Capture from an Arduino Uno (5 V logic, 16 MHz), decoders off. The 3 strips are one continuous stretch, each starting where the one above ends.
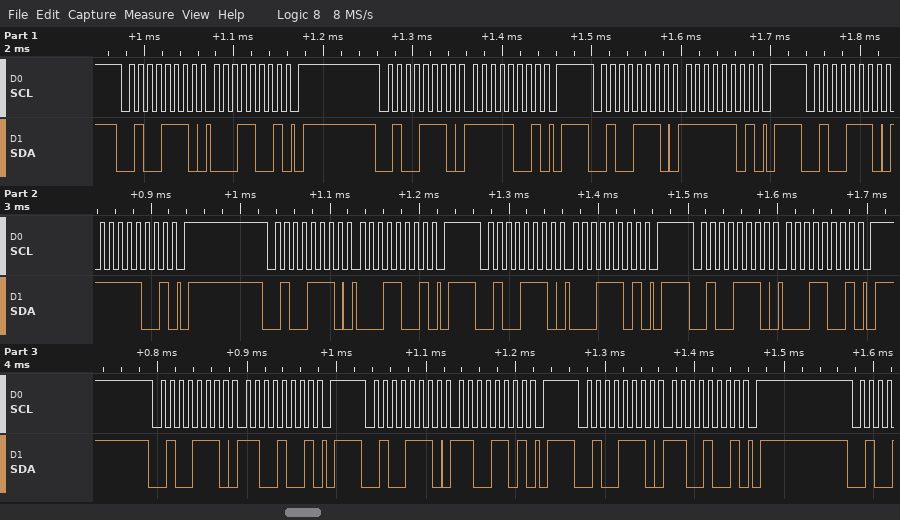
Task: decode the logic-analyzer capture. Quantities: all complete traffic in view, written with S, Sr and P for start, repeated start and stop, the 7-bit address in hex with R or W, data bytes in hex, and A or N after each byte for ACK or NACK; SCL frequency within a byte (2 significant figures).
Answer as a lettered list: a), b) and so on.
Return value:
a) S 27W A 19 A P S 27W A F9 A P S 27W A FD A P S 27W A F9 A P S 27W A 19 A P S 27W A 1D A P S 27W A 19 A P S 27W A C9 A P S 27W A CD A P S 27W A C9 A P
b) 100 kHz
